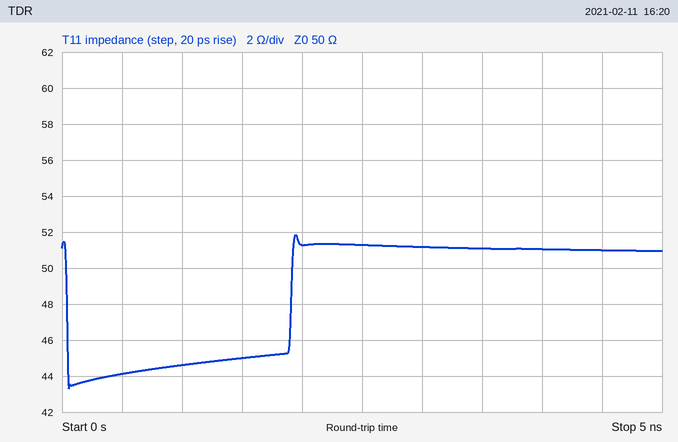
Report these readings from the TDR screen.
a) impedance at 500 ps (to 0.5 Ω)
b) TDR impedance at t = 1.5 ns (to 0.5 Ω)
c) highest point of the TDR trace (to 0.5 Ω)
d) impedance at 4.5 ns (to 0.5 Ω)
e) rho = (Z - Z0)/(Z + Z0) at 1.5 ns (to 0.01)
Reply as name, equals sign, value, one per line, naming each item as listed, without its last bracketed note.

impedance at 500 ps = 44.0 Ω
TDR impedance at t = 1.5 ns = 45.0 Ω
highest point of the TDR trace = 52.0 Ω
impedance at 4.5 ns = 51.0 Ω
rho = (Z - Z0)/(Z + Z0) at 1.5 ns = -0.05
